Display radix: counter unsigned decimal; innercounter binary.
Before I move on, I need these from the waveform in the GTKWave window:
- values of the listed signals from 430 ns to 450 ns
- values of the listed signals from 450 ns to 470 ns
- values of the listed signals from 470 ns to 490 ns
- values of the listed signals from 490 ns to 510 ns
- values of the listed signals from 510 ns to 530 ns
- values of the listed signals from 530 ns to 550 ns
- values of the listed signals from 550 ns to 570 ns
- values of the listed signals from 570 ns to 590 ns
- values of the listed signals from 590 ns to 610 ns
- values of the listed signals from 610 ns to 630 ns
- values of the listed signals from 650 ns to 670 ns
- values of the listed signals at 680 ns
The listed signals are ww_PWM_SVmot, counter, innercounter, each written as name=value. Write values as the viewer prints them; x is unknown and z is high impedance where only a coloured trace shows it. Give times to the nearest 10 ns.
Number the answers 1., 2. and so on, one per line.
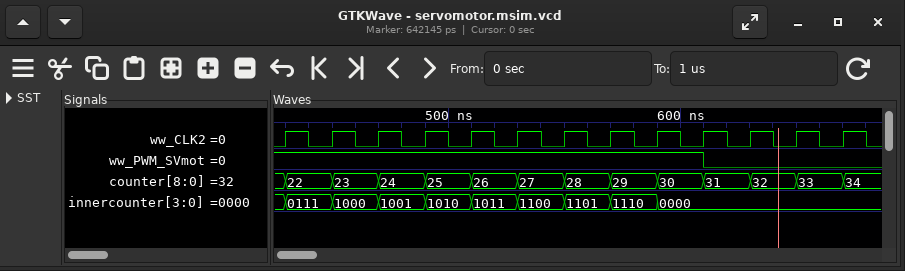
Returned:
1. ww_PWM_SVmot=1, counter=22, innercounter=0111
2. ww_PWM_SVmot=1, counter=23, innercounter=1000
3. ww_PWM_SVmot=1, counter=24, innercounter=1001
4. ww_PWM_SVmot=1, counter=25, innercounter=1010
5. ww_PWM_SVmot=1, counter=26, innercounter=1011
6. ww_PWM_SVmot=1, counter=27, innercounter=1100
7. ww_PWM_SVmot=1, counter=28, innercounter=1101
8. ww_PWM_SVmot=1, counter=29, innercounter=1110
9. ww_PWM_SVmot=1, counter=30, innercounter=0000
10. ww_PWM_SVmot=0, counter=31, innercounter=0000
11. ww_PWM_SVmot=0, counter=33, innercounter=0000
12. ww_PWM_SVmot=0, counter=34, innercounter=0000
